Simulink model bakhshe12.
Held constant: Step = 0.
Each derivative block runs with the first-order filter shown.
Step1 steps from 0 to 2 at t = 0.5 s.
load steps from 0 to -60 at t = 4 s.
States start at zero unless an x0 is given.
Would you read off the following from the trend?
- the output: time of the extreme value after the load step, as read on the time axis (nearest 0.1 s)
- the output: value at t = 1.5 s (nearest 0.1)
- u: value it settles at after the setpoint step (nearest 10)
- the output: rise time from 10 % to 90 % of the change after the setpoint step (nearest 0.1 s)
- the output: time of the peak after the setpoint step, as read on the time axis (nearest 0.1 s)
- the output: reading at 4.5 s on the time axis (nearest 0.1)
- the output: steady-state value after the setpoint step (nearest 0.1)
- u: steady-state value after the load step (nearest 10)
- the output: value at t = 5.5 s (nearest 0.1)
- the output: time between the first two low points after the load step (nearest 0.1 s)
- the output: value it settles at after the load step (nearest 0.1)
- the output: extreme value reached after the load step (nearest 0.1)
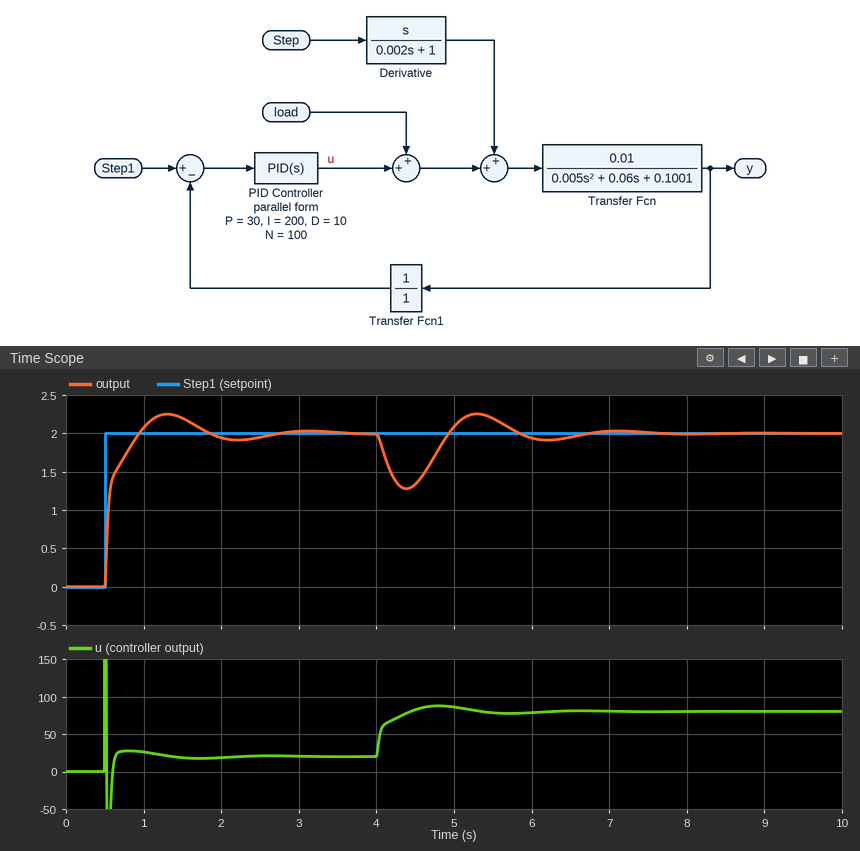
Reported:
4.4 s
2.2
20
0.3 s
1.3 s
1.3
2.0
80
2.2
1.8 s
2.0
1.3
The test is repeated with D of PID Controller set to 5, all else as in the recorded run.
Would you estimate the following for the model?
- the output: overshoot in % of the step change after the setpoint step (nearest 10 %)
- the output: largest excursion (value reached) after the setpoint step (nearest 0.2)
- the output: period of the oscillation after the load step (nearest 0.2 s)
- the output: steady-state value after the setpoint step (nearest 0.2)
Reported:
20 %
2.4
1.4 s
2.0
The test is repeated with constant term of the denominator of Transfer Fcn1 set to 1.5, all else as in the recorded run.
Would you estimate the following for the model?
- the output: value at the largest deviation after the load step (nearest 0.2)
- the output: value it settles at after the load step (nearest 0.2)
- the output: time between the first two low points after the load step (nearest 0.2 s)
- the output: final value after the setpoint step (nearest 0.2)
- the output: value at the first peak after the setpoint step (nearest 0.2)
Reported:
2.0
3.0
2.0 s
3.0
3.4
